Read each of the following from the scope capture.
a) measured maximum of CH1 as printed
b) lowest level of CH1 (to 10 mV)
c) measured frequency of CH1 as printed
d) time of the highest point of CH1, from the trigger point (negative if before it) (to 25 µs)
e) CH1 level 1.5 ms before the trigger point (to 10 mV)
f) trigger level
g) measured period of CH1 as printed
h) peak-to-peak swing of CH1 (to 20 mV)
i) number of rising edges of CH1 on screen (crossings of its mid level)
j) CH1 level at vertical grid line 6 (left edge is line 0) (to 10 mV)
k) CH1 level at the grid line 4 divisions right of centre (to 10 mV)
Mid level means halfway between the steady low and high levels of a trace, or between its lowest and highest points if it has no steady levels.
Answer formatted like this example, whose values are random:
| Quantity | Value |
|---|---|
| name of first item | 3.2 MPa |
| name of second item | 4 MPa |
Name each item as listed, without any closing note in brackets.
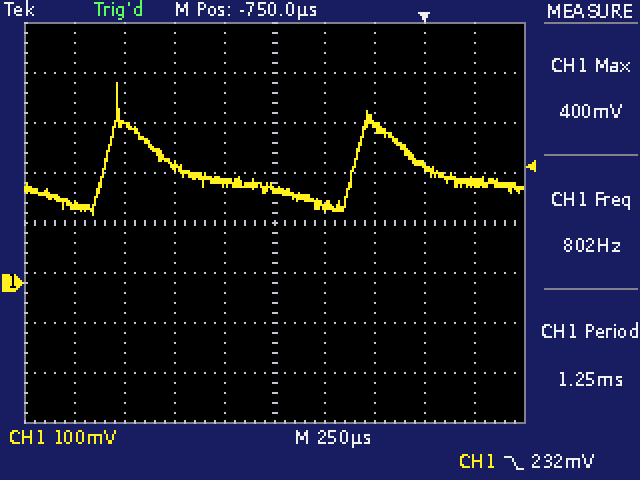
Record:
| Quantity | Value |
|---|---|
| measured maximum of CH1 as printed | 400 mV |
| lowest level of CH1 | 140 mV |
| measured frequency of CH1 as printed | 802 Hz |
| time of the highest point of CH1, from the trigger point (negative if before it) | -1.525 ms |
| CH1 level 1.5 ms before the trigger point | 320 mV |
| trigger level | 232 mV |
| measured period of CH1 as printed | 1.25 ms |
| peak-to-peak swing of CH1 | 260 mV |
| number of rising edges of CH1 on screen | 2 |
| CH1 level at vertical grid line 6 (left edge is line 0) | 150 mV |
| CH1 level at the grid line 4 divisions right of centre | 200 mV |
